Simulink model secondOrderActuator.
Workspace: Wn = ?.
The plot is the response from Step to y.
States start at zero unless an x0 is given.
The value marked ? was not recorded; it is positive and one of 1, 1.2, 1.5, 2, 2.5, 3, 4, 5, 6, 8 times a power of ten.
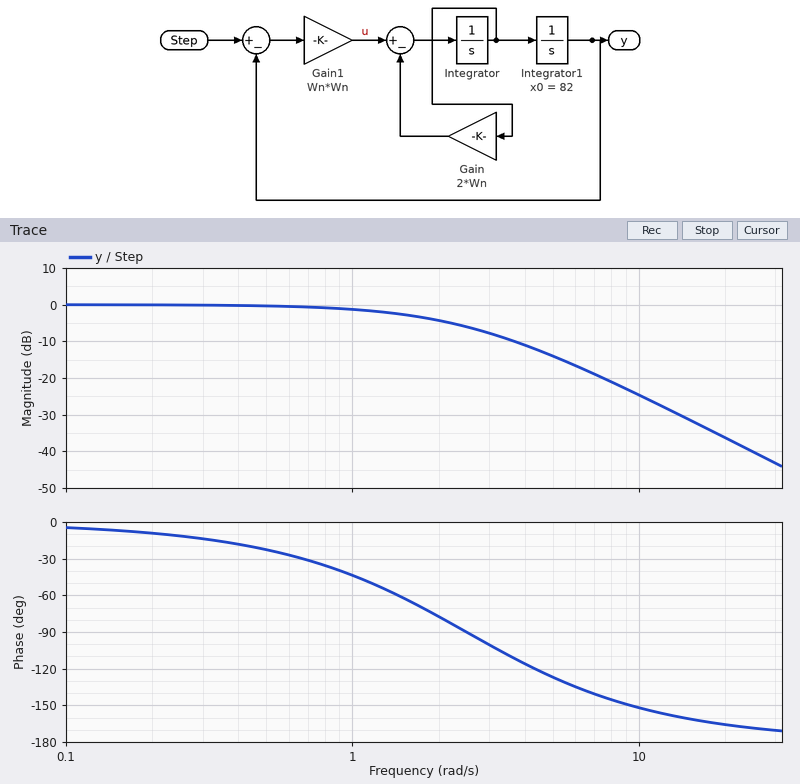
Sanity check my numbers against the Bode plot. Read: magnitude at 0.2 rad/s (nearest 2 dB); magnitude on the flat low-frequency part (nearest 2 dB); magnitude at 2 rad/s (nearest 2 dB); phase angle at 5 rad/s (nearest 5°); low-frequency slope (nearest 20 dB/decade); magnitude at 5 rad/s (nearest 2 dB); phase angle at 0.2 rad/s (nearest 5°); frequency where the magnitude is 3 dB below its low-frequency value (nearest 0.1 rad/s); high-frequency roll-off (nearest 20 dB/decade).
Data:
0 dB
0 dB
-4 dB
-125°
0 dB/decade
-14 dB
-10°
1.6 rad/s
-40 dB/decade
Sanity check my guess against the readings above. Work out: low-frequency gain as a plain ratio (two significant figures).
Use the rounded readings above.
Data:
1.0
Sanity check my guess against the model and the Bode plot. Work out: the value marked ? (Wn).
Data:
2.5
